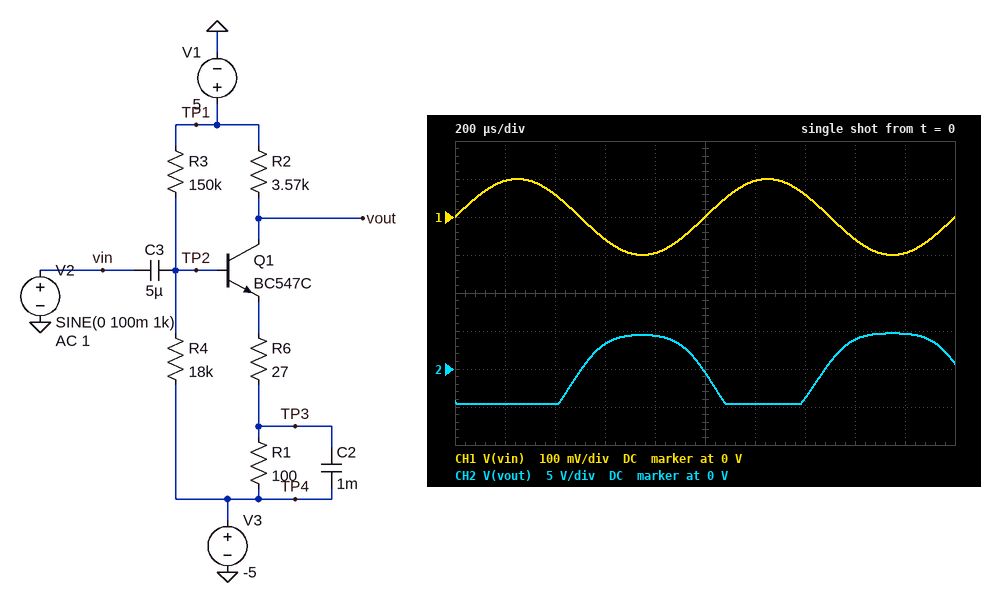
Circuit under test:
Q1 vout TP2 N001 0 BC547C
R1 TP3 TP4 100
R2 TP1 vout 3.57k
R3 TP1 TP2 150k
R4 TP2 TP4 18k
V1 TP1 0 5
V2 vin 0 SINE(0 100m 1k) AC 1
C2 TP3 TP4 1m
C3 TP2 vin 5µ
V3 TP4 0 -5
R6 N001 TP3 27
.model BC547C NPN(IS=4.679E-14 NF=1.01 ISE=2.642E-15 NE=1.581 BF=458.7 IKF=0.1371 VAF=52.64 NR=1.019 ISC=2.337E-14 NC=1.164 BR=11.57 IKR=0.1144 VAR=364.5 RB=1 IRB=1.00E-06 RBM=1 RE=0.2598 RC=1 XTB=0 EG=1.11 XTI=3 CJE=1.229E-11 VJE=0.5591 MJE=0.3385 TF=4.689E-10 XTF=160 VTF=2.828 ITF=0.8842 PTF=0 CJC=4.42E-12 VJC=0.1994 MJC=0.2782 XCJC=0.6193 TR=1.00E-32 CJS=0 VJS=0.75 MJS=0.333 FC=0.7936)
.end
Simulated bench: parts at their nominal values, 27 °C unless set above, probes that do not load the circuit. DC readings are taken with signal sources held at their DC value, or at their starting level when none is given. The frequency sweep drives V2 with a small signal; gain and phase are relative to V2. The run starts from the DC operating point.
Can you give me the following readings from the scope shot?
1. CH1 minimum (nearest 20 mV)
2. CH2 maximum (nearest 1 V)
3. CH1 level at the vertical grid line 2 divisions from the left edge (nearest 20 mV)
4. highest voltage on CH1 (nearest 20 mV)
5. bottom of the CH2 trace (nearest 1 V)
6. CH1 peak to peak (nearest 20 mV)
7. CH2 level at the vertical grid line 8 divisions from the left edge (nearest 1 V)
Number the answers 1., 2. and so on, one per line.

1. -100 mV
2. 5 V
3. 60 mV
4. 100 mV
5. -5 V
6. 200 mV
7. 4 V
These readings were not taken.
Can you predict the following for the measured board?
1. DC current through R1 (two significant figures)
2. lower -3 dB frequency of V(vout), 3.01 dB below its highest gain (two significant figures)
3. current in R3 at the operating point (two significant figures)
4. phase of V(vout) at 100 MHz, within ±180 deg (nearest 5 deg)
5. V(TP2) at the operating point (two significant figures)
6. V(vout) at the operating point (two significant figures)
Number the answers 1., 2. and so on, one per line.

1. 2.6 mA
2. 8.1 Hz
3. 60 µA
4. 60 deg
5. -4.0 V
6. -4.3 V
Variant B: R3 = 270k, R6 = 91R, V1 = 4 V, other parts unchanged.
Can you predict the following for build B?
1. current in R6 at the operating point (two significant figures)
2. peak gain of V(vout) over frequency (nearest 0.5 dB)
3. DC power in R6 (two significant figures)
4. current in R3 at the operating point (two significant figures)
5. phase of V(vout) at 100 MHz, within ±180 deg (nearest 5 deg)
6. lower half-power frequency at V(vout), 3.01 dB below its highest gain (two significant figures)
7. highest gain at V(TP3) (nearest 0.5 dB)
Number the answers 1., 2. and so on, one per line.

1. 68 µA
2. 17.5 dB
3. 420 nW
4. 31 µA
5. 35 deg
6. 2.3 Hz
7. -21.5 dB
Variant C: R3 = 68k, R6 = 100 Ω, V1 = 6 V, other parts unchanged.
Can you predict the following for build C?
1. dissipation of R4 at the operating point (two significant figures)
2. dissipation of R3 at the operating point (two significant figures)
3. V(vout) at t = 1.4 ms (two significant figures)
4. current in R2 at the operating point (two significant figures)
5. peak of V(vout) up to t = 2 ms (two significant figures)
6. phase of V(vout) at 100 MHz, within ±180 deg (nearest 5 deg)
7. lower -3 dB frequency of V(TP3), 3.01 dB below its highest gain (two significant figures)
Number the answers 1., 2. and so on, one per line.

1. 87 µW
2. 1.4 mW
3. -4.4 V
4. 2.9 mA
5. -350 mV
6. 20 deg
7. 1.6 Hz
